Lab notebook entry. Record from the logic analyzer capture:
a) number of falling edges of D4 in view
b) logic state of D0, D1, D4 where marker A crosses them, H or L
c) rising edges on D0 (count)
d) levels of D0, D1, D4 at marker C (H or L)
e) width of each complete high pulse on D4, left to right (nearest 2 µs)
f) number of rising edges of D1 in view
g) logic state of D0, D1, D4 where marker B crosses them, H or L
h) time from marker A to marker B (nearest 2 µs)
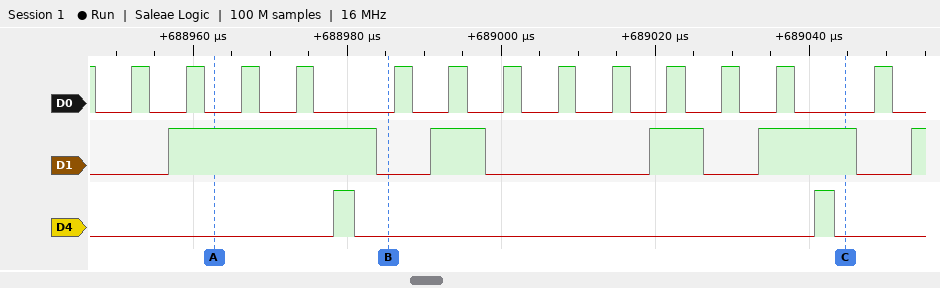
2
D0=L, D1=H, D4=L
13
D0=L, D1=H, D4=L
2 µs, 2 µs
5
D0=L, D1=L, D4=L
22 µs
